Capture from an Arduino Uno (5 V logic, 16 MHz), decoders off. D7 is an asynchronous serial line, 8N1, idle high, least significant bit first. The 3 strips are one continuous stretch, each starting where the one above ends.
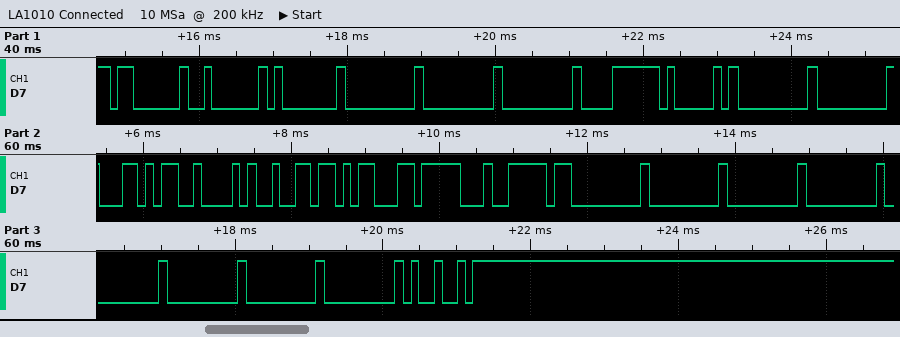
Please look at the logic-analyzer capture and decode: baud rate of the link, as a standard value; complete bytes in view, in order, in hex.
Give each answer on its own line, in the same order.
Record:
9600 baud
03 02 01 00 00 00 F8 41 00 00 AC 42 B2 8D 1F BE 00 00 00 00 00 00 00 00 49
